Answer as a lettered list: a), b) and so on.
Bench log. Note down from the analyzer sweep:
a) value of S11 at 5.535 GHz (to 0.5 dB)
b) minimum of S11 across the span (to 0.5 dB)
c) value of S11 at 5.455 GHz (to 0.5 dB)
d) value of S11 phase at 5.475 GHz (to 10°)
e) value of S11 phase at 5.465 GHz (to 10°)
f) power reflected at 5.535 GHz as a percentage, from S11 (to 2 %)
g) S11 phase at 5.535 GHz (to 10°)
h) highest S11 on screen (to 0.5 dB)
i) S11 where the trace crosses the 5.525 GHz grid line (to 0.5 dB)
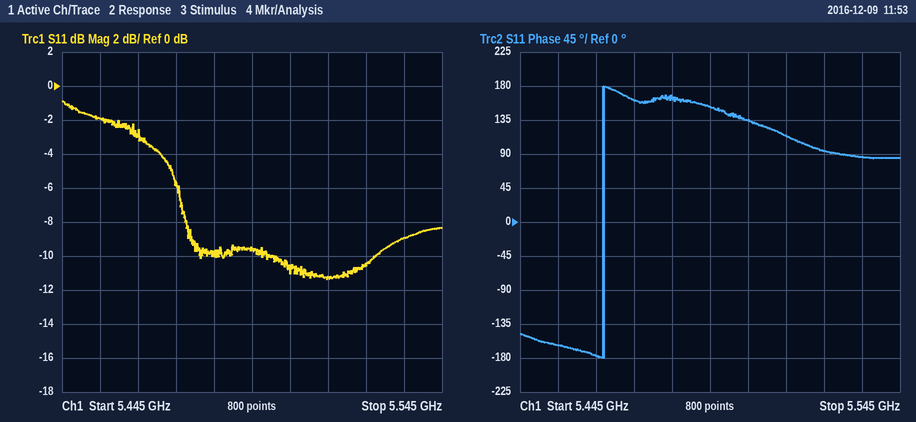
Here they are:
a) -9.0 dB
b) -11.5 dB
c) -2.0 dB
d) 160°
e) -180°
f) 12 %
g) 90°
h) -1.0 dB
i) -10.5 dB
